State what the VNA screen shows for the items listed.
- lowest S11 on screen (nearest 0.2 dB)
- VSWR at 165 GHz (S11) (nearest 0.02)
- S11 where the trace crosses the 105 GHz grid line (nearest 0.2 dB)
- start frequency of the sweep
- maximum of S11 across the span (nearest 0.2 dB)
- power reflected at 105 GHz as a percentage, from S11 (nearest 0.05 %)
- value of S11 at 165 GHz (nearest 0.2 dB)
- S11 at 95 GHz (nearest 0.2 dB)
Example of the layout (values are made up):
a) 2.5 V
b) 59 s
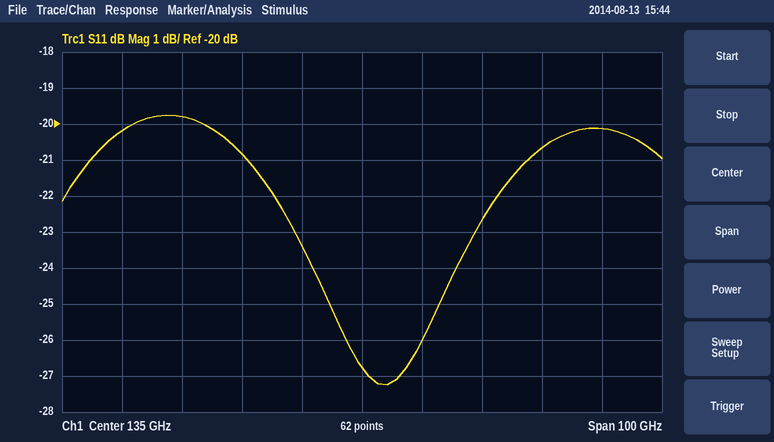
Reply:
a) -27.2 dB
b) 1.20
c) -19.8 dB
d) 85 GHz
e) -19.8 dB
f) 1.05 %
g) -20.6 dB
h) -20.2 dB
